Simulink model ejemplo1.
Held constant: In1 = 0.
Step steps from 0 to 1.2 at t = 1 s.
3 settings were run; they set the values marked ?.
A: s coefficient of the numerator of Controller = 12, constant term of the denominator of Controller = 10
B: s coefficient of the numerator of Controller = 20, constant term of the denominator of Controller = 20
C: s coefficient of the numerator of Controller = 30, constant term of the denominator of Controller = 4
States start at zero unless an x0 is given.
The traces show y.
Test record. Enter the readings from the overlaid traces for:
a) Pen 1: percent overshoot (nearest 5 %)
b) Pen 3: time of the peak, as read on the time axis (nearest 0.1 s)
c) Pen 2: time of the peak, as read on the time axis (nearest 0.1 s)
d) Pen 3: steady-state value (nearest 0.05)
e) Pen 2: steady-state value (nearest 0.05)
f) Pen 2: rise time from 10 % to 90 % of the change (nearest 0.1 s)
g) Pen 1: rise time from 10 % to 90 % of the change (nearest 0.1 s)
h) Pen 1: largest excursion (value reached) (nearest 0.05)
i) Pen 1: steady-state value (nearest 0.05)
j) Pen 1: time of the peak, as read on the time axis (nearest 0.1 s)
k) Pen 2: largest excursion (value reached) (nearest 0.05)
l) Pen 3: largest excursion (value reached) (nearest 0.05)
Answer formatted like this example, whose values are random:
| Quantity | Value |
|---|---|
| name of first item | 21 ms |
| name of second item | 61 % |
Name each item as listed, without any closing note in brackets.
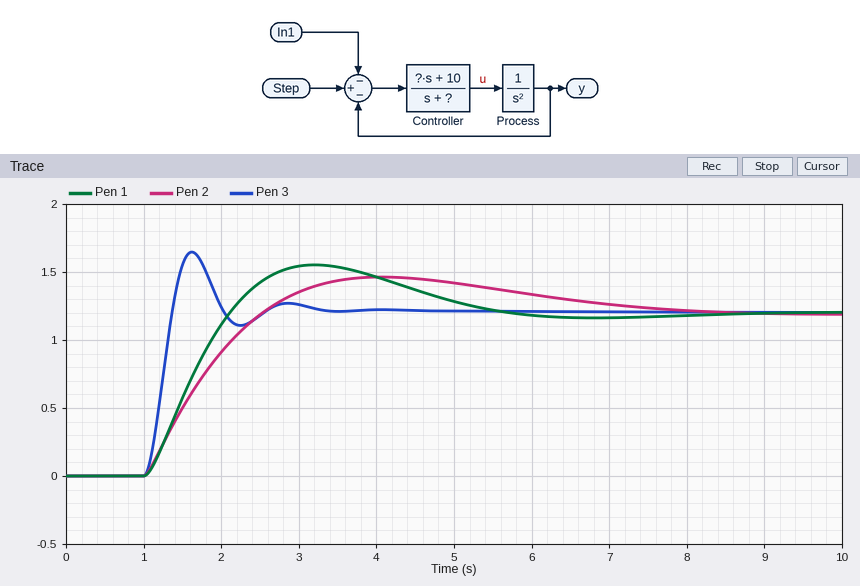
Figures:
| Quantity | Value |
|---|---|
| Pen 1: percent overshoot | 30 % |
| Pen 3: time of the peak, as read on the time axis | 1.6 s |
| Pen 2: time of the peak, as read on the time axis | 4.1 s |
| Pen 3: steady-state value | 1.20 |
| Pen 2: steady-state value | 1.20 |
| Pen 2: rise time from 10 % to 90 % of the change | 1.1 s |
| Pen 1: rise time from 10 % to 90 % of the change | 0.8 s |
| Pen 1: largest excursion (value reached) | 1.55 |
| Pen 1: steady-state value | 1.20 |
| Pen 1: time of the peak, as read on the time axis | 3.2 s |
| Pen 2: largest excursion (value reached) | 1.45 |
| Pen 3: largest excursion (value reached) | 1.65 |
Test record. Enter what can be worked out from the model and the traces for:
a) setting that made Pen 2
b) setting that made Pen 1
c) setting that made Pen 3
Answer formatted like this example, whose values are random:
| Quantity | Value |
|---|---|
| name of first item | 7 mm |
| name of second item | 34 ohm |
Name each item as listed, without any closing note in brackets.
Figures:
| Quantity | Value |
|---|---|
| setting that made Pen 2 | B |
| setting that made Pen 1 | A |
| setting that made Pen 3 | C |
